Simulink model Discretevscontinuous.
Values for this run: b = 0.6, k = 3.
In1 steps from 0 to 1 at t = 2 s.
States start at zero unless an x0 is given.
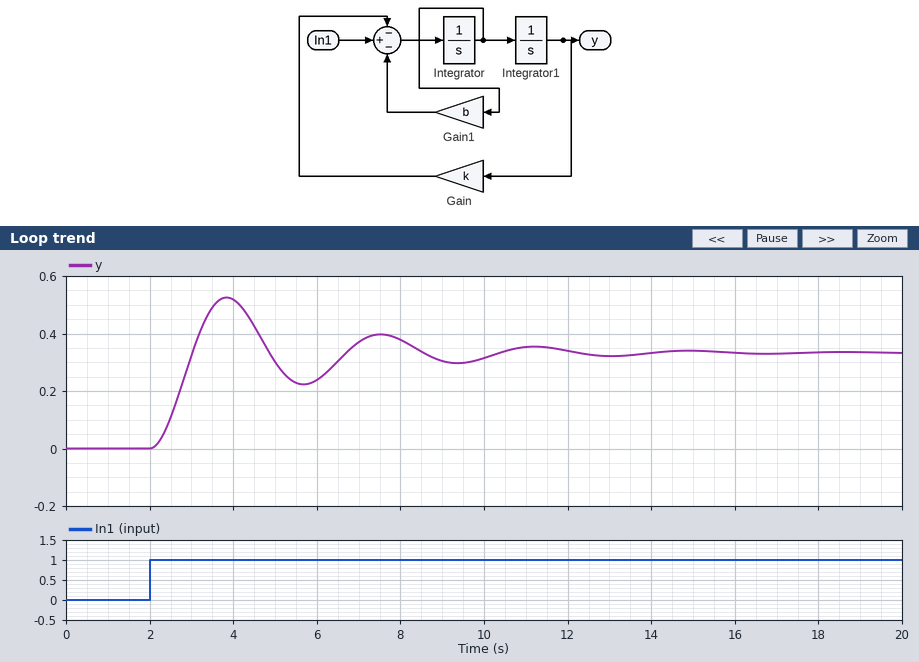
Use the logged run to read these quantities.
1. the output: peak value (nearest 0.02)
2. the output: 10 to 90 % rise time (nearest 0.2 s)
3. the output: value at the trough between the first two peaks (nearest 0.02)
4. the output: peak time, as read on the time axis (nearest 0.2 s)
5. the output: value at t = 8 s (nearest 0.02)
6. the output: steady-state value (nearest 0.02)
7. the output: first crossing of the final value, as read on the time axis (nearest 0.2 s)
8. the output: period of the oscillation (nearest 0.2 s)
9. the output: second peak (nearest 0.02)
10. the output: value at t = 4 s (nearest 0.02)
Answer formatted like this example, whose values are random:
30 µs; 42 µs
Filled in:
0.52; 0.6 s; 0.22; 3.8 s; 0.38; 0.34; 3.0 s; 3.6 s; 0.40; 0.52
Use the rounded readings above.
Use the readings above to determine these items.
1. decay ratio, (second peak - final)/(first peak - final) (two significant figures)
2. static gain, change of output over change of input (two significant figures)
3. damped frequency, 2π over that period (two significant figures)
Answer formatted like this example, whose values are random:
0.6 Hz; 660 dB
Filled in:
0.33; 0.34; 1.7 rad/s
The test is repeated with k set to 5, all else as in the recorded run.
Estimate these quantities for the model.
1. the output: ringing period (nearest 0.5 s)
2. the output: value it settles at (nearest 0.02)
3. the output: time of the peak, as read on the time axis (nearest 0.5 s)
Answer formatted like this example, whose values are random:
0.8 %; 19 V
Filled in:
3.0 s; 0.20; 3.5 s
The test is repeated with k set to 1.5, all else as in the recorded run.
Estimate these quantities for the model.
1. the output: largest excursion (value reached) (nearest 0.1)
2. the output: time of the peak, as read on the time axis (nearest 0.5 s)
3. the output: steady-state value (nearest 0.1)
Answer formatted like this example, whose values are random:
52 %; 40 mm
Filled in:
1.0; 4.5 s; 0.7
